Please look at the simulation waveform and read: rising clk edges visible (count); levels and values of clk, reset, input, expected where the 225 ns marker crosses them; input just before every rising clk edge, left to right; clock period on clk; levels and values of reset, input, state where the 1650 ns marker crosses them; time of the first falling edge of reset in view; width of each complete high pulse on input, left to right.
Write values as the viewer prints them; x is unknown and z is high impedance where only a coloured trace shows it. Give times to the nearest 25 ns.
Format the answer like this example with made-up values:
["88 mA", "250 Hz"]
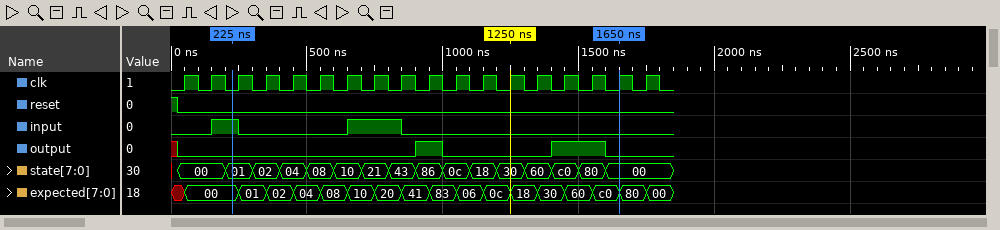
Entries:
["18", "clk=0, reset=0, input=1, expected=00", "0 0 1 0 0 0 0 1 1 0 0 0 0 0 0 0 0 0", "100 ns", "reset=0, input=0, state=00", "25 ns", "100 ns, 200 ns"]
